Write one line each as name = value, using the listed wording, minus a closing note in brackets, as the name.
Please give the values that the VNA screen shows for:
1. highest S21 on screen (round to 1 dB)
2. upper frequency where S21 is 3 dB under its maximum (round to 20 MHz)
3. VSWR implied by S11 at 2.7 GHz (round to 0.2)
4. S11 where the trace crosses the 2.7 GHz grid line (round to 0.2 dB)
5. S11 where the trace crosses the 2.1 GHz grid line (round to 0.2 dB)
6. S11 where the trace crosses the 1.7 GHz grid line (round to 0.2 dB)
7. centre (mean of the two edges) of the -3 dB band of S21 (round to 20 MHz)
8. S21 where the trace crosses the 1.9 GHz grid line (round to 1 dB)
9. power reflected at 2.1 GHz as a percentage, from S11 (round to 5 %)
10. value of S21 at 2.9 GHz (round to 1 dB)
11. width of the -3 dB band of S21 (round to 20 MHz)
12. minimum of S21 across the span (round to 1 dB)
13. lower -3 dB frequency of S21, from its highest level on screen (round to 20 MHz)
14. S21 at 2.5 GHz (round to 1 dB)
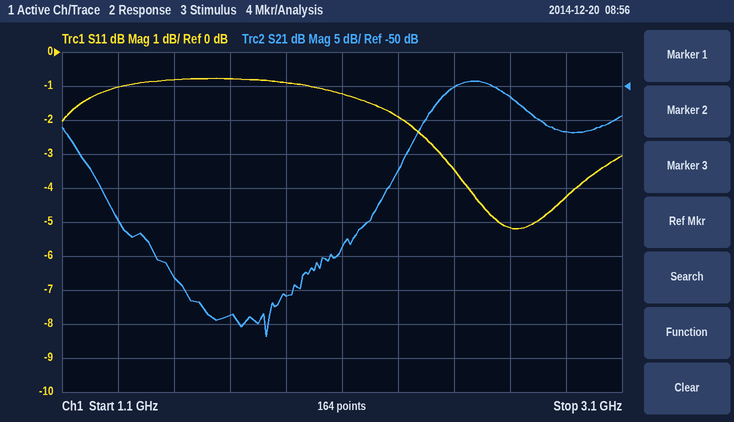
highest S21 on screen = -49 dB
upper frequency where S21 is 3 dB under its maximum = 2.72 GHz
VSWR implied by S11 at 2.7 GHz = 3.4
S11 where the trace crosses the 2.7 GHz grid line = -5.2 dB
S11 where the trace crosses the 2.1 GHz grid line = -1.2 dB
S11 where the trace crosses the 1.7 GHz grid line = -0.8 dB
centre (mean of the two edges) of the -3 dB band of S21 = 2.58 GHz
S21 where the trace crosses the 1.9 GHz grid line = -81 dB
power reflected at 2.1 GHz as a percentage, from S11 = 75 %
value of S21 at 2.9 GHz = -57 dB
width of the -3 dB band of S21 = 280 MHz
minimum of S21 across the span = -87 dB
lower -3 dB frequency of S21, from its highest level on screen = 2.44 GHz
S21 at 2.5 GHz = -50 dB
